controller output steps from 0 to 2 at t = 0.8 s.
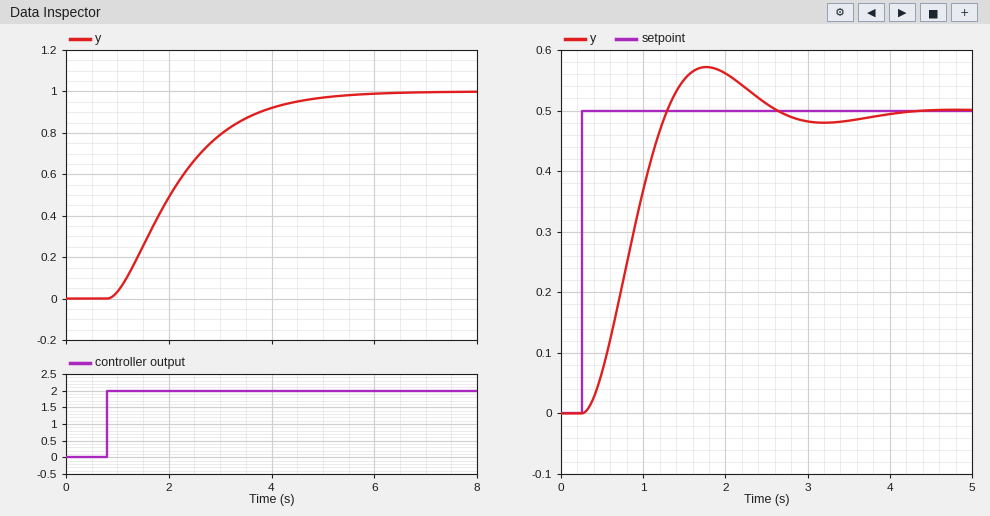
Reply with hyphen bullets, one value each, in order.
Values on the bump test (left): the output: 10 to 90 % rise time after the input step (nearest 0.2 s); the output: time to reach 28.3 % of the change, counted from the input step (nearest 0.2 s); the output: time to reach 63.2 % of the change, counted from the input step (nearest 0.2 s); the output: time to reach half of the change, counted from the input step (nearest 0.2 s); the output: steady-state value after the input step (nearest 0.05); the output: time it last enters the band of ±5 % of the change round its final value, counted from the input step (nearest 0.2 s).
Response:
- 2.6 s
- 0.8 s
- 1.6 s
- 1.2 s
- 1.00
- 3.6 s
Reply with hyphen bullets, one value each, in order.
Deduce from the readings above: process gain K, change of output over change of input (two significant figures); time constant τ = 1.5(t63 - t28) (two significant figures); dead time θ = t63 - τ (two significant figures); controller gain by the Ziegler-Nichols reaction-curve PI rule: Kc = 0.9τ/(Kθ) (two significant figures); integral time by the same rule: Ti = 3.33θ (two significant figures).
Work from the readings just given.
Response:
- 0.50
- 1.2 s
- 0.40 s
- 5.4
- 1.3 s
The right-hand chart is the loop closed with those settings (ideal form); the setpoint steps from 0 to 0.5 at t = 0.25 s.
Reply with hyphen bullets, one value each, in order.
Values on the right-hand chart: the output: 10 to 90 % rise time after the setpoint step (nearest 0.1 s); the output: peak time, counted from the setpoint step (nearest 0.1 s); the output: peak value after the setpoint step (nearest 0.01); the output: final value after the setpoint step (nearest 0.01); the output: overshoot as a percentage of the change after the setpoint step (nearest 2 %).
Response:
- 0.7 s
- 1.5 s
- 0.57
- 0.50
- 14 %
